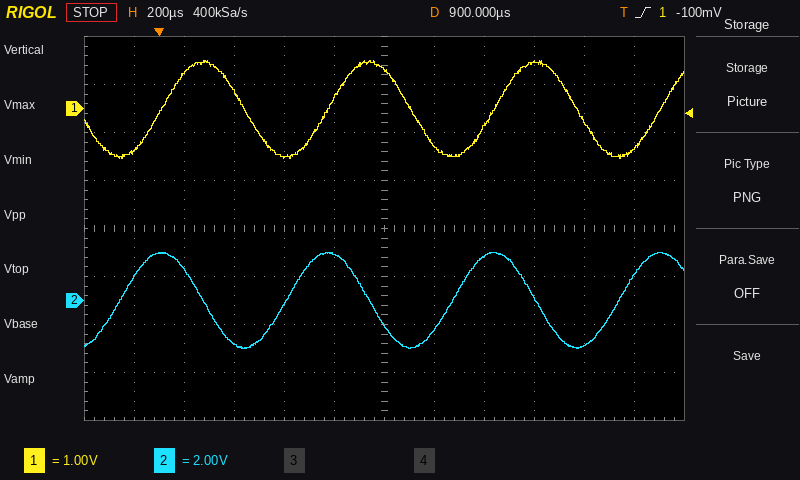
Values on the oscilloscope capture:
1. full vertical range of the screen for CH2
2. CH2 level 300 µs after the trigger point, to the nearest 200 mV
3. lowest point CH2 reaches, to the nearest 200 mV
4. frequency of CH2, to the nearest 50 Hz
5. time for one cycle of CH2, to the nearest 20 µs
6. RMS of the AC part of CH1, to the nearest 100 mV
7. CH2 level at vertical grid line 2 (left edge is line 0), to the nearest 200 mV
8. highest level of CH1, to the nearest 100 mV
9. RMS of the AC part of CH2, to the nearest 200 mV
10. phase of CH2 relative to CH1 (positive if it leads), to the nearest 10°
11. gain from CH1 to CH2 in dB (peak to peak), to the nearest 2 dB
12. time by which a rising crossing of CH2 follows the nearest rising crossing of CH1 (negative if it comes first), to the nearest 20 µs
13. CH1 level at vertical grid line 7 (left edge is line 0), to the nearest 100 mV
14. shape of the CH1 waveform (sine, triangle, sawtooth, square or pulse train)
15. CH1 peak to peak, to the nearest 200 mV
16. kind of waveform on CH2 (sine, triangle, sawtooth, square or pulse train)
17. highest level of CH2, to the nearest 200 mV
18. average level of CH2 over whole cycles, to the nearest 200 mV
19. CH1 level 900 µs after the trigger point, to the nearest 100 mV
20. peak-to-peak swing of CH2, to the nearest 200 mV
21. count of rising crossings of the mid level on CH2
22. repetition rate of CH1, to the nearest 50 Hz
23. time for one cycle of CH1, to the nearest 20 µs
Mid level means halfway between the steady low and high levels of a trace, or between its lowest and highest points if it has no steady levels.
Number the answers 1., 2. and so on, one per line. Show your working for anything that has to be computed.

1. 16 V
2. -1.8 V
3. -2.0 V
4. 1 / 660 µs ≈ 1.52 kHz, so 1.50 kHz to the nearest 50 Hz
5. 660 µs
6. 2.0 V / (2√2) ≈ 707 mV, so 700 mV to the nearest 100 mV
7. 1.2 V
8. 1.0 V
9. 4.0 V / (2√2) ≈ 1.4 V
10. −360° × (-160 µs) / 660 µs ≈ +87.3°, so +90° to the nearest 10°
11. 20 log10(4.0 V / 2.0 V) ≈ 6 dB
12. -160 µs
13. -800 mV
14. sine
15. 2.0 V
16. sine
17. 2.0 V
18. (2.0 V + (-2.0 V)) / 2 ≈ 0.0 V
19. 800 mV
20. 2.0 V − (-2.0 V) = 4.0 V
21. 4
22. 1 / 660 µs ≈ 1.52 kHz, so 1.50 kHz to the nearest 50 Hz
23. 660 µs
